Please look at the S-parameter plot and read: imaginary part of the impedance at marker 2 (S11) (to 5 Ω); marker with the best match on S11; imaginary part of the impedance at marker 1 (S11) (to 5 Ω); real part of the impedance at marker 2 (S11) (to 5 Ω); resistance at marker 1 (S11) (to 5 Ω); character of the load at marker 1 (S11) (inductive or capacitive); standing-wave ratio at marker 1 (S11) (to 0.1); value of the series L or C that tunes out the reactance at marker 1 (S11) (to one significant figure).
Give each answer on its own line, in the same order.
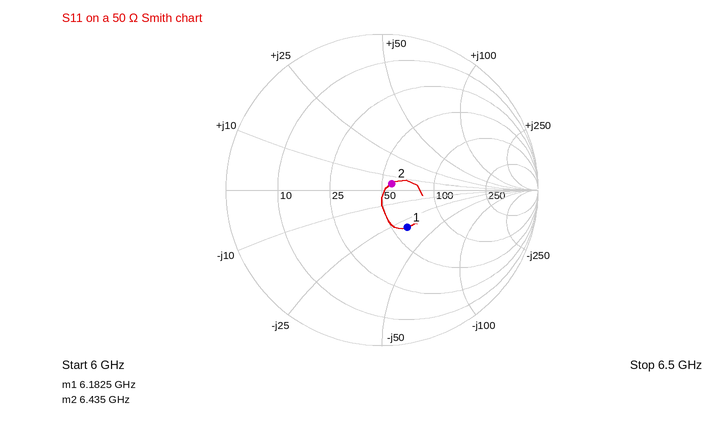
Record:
+5 Ω
marker 2
-30 Ω
55 Ω
60 Ω
capacitive
1.8
800 pH
